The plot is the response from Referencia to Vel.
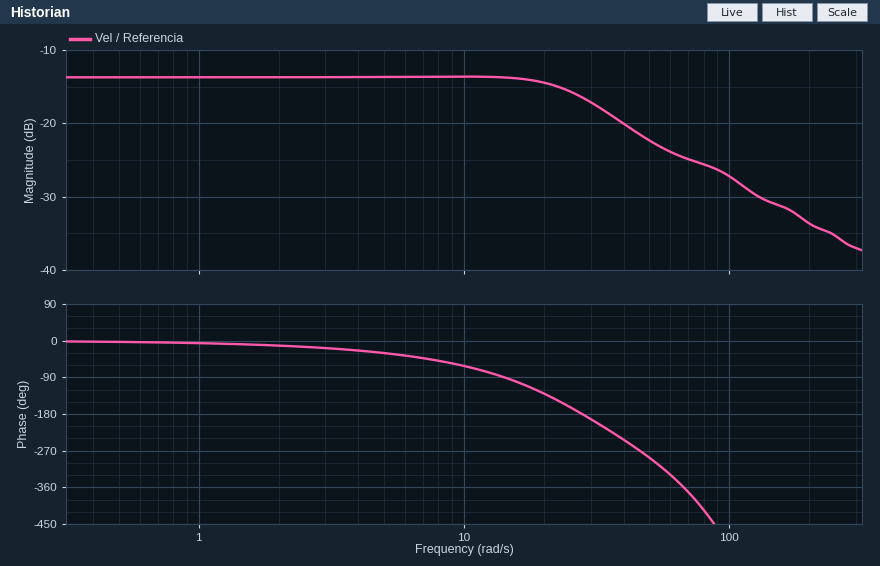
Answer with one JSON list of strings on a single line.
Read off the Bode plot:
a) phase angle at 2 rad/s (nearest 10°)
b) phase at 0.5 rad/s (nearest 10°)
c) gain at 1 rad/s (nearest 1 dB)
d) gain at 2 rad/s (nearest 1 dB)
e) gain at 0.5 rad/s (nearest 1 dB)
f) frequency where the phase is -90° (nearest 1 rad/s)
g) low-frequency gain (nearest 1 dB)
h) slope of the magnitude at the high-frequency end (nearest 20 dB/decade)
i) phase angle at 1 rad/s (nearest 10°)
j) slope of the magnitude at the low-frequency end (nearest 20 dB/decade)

["-10°", "0°", "-14 dB", "-14 dB", "-14 dB", "14 rad/s", "-14 dB", "-20 dB/decade", "-10°", "0 dB/decade"]
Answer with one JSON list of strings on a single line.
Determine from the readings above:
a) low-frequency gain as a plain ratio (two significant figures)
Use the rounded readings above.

["0.20"]
